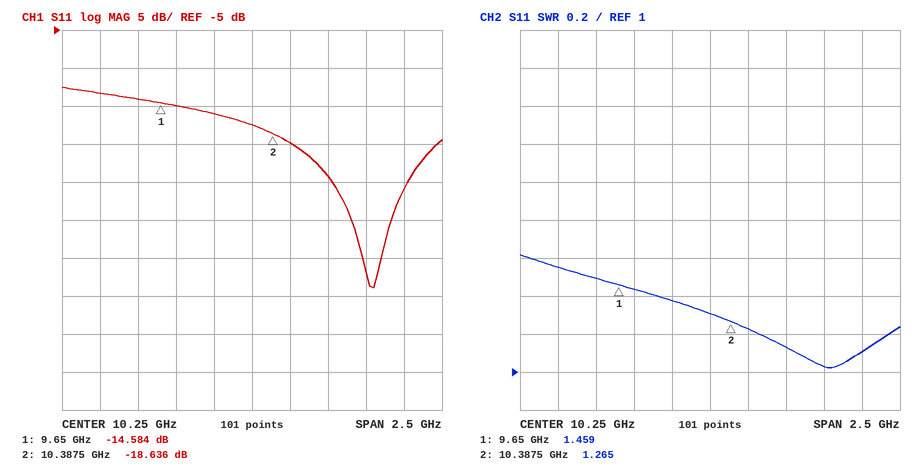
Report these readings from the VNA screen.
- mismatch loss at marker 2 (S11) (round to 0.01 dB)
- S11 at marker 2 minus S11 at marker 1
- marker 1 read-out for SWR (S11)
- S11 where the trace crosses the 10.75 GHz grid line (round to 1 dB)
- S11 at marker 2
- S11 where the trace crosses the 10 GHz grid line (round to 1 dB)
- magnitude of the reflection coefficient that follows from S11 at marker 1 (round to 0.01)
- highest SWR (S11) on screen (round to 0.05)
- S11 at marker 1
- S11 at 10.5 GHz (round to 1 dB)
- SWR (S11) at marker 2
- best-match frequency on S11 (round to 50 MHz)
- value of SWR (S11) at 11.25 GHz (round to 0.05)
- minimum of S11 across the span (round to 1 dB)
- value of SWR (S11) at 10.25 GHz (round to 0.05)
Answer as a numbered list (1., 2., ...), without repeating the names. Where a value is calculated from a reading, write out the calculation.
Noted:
1. −10 log10(1 − 10^(-18.636/10)) ≈ 0.06 dB
2. -18.636 − (-14.584) = -4.052 dB
3. 1.459
4. -24 dB
5. -18.636 dB
6. -16 dB
7. 10^(-14.584/20) ≈ 0.19
8. 1.60
9. -14.584 dB
10. -20 dB
11. 1.265
12. 11.05 GHz
13. 1.10
14. -39 dB
15. 1.30
